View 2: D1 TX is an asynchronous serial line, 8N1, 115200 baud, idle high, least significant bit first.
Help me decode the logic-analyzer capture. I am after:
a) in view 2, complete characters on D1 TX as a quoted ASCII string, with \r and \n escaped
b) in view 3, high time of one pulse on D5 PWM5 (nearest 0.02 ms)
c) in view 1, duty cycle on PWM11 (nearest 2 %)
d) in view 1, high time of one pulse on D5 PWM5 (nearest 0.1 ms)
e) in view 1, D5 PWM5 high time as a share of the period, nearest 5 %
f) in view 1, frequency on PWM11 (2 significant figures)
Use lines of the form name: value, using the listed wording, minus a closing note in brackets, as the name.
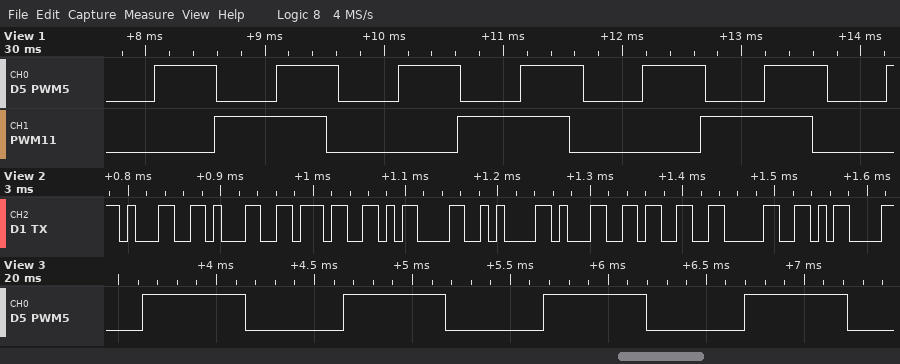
in view 2, complete characters on D1 TX as a quoted ASCII string, with \r and \n escaped: "117\r\n130\r"
in view 3, high time of one pulse on D5 PWM5: 0.52 ms
in view 1, duty cycle on PWM11: 46 %
in view 1, high time of one pulse on D5 PWM5: 0.5 ms
in view 1, D5 PWM5 high time as a share of the period, nearest 5 %: 50 %
in view 1, frequency on PWM11: 490 Hz
